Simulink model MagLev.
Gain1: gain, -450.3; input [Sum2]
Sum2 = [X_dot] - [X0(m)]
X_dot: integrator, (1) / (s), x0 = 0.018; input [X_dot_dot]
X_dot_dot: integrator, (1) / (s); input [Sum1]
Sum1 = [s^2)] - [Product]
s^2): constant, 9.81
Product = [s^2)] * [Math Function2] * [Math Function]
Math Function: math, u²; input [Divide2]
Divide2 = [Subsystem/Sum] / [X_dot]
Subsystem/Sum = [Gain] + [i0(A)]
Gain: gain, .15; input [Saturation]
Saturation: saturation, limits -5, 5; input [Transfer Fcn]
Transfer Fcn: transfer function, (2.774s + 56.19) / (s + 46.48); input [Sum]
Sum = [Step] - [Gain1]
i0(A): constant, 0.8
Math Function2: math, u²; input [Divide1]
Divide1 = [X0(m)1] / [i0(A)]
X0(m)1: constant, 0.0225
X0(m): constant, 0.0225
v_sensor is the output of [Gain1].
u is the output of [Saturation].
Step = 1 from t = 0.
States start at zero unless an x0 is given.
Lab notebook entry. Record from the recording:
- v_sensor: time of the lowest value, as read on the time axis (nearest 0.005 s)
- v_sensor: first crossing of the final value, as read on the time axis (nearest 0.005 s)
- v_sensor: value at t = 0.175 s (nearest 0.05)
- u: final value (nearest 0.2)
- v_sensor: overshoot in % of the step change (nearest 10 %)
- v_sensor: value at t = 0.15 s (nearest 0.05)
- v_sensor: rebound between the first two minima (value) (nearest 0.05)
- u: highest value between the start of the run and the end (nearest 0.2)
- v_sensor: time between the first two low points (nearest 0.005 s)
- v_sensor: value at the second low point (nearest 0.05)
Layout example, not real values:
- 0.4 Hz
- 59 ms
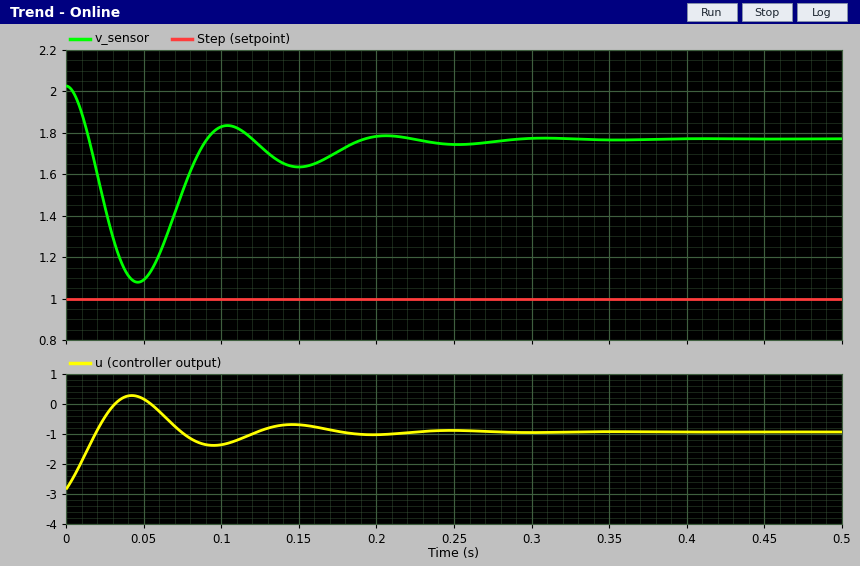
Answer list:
- 0.045 s
- 0.015 s
- 1.70
- -1.0
- 270 %
- 1.65
- 1.85
- 0.2
- 0.105 s
- 1.65
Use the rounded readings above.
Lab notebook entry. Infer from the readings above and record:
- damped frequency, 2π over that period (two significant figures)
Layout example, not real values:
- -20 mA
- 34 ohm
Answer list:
- 60 rad/s
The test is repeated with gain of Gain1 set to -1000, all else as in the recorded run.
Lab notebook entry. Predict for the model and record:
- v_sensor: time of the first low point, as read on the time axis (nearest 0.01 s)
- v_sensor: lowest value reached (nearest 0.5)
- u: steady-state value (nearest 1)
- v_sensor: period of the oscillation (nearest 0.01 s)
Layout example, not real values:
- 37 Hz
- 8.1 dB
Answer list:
- 0.04 s
- 0.0
- 0
- 0.07 s
